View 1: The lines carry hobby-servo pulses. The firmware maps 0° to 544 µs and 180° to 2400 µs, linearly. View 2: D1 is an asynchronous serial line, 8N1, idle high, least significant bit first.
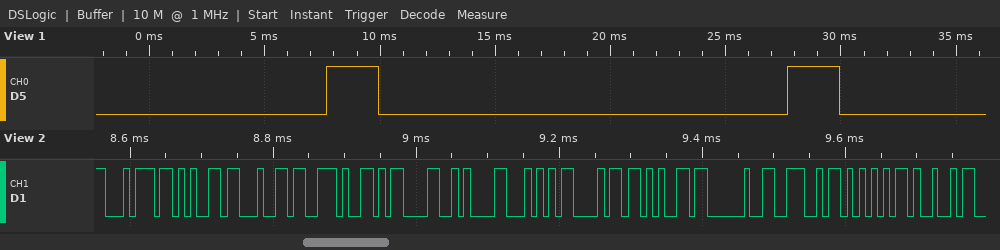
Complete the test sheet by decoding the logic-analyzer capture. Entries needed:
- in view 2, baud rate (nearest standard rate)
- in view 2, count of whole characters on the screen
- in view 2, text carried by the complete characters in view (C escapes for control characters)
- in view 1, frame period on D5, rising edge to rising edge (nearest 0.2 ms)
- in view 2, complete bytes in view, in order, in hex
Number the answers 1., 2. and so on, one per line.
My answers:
1. 115200 baud
2. 13
3. "ted.\r\nThe NUI"
4. 20.0 ms
5. 74 65 64 2E 0D 0A 54 68 65 20 4E 55 49
